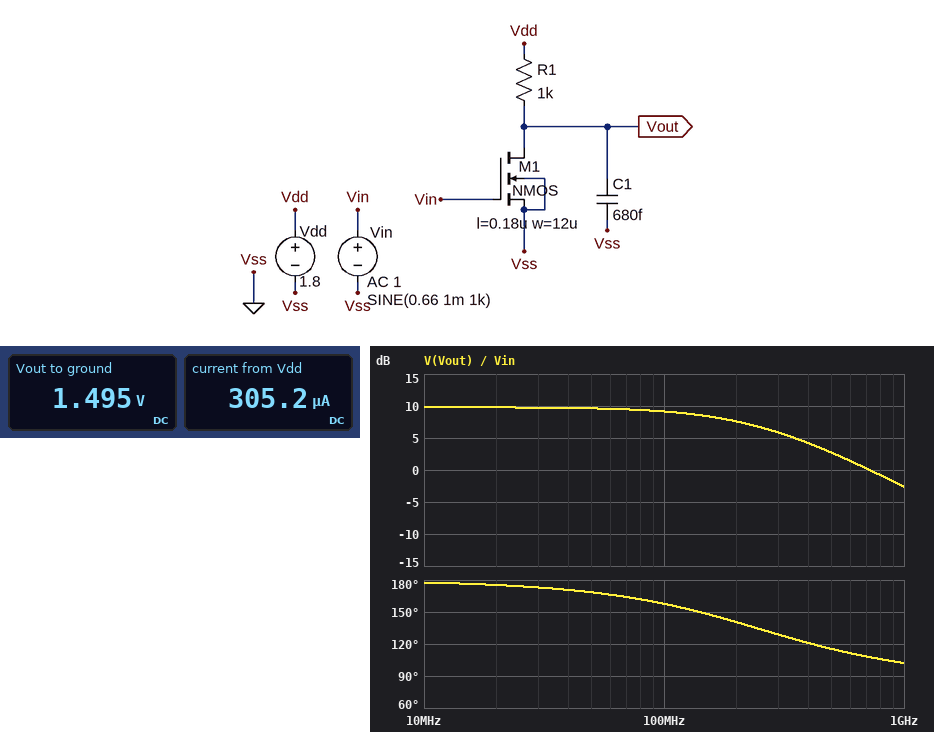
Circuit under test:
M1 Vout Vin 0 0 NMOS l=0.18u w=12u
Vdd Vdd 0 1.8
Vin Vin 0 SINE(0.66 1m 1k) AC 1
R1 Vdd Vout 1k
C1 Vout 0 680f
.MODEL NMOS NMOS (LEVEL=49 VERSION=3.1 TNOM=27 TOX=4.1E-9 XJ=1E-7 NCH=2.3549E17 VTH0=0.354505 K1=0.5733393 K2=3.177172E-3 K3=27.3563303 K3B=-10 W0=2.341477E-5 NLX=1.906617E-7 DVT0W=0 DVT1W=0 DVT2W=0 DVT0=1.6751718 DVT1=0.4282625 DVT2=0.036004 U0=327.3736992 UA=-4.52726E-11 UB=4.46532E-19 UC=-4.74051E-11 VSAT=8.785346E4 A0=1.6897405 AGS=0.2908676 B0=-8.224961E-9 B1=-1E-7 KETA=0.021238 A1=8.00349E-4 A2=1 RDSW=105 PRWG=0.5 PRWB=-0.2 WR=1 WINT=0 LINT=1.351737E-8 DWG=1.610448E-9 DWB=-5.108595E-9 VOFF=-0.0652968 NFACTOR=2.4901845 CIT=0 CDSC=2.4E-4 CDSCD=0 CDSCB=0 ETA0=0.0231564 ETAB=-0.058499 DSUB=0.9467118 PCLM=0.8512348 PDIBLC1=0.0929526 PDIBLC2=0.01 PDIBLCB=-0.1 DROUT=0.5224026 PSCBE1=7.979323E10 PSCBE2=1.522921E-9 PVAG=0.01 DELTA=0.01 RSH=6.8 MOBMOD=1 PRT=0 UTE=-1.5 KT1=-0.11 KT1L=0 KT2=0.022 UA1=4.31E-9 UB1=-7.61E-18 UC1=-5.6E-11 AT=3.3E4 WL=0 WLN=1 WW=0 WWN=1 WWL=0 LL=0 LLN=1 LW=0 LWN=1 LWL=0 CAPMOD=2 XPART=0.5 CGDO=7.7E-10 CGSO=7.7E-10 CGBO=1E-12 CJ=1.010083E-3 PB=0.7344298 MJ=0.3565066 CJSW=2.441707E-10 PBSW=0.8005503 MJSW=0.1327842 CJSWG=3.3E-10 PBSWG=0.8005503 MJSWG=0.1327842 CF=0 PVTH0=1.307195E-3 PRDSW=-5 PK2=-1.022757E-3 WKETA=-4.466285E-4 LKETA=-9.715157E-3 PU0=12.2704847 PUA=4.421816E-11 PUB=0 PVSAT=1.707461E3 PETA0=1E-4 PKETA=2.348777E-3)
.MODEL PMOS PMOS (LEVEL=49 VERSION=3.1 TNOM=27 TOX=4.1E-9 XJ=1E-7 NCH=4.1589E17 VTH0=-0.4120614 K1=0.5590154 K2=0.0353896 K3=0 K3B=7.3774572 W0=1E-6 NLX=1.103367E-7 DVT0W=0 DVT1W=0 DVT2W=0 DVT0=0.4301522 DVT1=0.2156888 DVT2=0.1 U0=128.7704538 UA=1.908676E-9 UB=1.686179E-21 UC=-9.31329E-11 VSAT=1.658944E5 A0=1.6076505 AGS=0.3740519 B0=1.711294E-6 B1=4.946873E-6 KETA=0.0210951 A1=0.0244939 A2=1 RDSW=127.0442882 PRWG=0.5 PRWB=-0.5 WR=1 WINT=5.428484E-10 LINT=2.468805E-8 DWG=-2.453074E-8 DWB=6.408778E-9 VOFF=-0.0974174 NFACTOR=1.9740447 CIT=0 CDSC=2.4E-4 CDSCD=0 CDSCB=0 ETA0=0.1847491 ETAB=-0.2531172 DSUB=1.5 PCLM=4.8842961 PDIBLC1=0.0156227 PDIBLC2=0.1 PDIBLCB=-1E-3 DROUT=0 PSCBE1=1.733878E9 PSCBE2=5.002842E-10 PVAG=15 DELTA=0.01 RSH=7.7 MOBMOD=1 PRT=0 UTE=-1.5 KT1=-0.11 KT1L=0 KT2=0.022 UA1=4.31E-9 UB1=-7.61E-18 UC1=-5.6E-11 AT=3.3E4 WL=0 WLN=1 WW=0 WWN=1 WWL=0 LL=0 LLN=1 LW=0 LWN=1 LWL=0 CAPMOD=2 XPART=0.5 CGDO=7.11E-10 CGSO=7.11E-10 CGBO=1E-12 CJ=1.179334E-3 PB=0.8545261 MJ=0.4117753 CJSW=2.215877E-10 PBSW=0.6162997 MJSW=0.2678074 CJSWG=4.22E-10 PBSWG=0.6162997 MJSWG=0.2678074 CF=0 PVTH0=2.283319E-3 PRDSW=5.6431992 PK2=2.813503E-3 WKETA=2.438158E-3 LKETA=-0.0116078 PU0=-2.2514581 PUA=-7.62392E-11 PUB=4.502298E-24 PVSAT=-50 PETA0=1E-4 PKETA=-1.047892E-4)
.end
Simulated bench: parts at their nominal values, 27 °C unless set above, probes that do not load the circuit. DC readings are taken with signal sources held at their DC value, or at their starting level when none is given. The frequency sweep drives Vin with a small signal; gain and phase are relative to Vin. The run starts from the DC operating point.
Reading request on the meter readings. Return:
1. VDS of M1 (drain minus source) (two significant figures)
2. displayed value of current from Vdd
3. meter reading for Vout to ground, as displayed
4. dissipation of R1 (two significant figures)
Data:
1.5 V
305.2 µA
1.495 V
93 µW
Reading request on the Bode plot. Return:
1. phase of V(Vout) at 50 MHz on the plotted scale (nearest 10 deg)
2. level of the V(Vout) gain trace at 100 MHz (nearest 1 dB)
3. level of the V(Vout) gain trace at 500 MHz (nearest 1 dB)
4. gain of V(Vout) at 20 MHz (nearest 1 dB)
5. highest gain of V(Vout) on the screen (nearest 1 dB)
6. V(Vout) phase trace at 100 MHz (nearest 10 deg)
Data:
170 deg
9 dB
3 dB
10 dB
10 dB
160 deg
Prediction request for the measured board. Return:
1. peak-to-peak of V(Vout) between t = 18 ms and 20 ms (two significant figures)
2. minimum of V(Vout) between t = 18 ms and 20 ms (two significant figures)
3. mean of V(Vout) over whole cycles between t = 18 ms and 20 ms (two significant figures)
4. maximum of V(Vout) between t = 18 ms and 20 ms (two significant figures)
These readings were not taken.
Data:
6.2 mV
1.5 V
1.5 V
1.5 V
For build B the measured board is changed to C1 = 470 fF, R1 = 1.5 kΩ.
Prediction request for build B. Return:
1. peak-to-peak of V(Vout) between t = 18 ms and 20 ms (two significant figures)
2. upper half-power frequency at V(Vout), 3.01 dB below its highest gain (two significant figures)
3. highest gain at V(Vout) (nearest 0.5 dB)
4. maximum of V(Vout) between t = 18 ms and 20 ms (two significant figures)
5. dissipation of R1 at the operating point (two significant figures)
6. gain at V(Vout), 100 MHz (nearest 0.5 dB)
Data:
8.8 mV
240 MHz
13.0 dB
1.4 V
130 µW
12.0 dB
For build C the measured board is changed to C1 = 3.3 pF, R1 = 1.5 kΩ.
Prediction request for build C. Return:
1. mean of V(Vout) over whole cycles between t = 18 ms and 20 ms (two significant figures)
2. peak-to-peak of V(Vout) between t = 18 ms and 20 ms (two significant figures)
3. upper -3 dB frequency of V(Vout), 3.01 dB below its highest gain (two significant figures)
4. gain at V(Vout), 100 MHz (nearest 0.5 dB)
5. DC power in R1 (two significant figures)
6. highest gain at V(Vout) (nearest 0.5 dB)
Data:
1.4 V
8.8 mV
35 MHz
3.5 dB
130 µW
13.0 dB
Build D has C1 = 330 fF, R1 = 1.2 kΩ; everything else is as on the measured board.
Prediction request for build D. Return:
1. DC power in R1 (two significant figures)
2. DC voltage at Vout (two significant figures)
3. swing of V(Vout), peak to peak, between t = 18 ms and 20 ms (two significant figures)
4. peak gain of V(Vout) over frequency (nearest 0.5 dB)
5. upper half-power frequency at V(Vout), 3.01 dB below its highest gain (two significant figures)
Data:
110 µW
1.4 V
7.3 mV
11.0 dB
420 MHz
